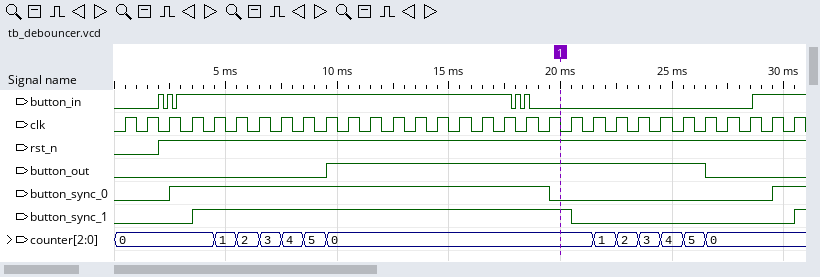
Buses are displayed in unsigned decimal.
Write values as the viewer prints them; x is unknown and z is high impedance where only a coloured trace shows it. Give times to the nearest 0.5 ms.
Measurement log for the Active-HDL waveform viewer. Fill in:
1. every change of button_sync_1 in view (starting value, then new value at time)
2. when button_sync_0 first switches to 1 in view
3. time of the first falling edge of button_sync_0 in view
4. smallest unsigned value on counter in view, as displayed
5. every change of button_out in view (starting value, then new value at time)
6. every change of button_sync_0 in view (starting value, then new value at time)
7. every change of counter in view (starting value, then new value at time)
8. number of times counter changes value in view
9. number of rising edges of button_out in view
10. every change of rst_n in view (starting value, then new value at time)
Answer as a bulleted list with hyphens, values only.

- 0, 1 at 3.5 ms, 0 at 20.5 ms, 1 at 30.5 ms
- 2.5 ms
- 19.5 ms
- 0
- 0, 1 at 9.5 ms, 0 at 26.5 ms
- 0, 1 at 2.5 ms, 0 at 19.5 ms, 1 at 29.5 ms
- 0, 1 at 4.5 ms, 2 at 5.5 ms, 3 at 6.5 ms, 4 at 7.5 ms, 5 at 8.5 ms, 0 at 9.5 ms, 1 at 21.5 ms, 2 at 22.5 ms, 3 at 23.5 ms, 4 at 24.5 ms, 5 at 25.5 ms, 0 at 26.5 ms
- 12
- 1
- 0, 1 at 2 ms
